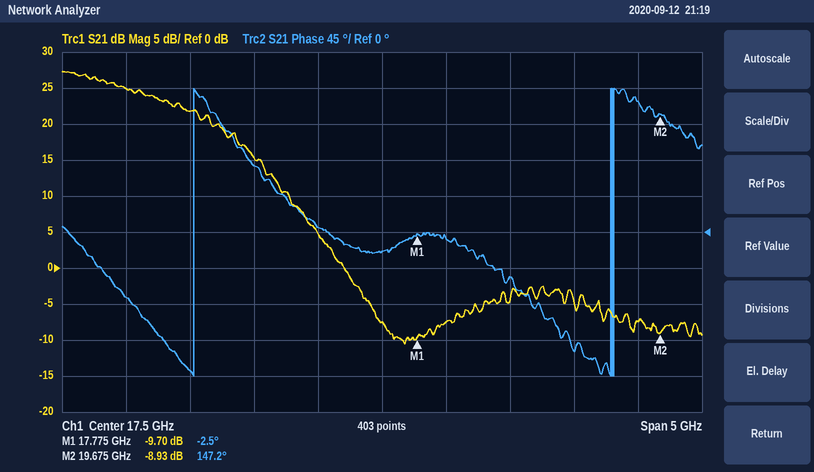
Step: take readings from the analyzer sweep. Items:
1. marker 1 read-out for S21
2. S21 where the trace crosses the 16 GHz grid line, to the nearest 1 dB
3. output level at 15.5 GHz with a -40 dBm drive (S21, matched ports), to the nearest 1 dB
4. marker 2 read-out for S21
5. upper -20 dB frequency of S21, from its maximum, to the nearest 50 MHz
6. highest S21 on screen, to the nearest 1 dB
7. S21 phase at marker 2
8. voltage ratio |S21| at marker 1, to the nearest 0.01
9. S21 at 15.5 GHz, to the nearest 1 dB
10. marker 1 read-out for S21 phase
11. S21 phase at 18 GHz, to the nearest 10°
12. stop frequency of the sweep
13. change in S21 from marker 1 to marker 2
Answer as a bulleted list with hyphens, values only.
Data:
- -9.70 dB
- 22 dB
- -15 dBm
- -8.93 dB
- 16.90 GHz
- 27 dB
- 147.2°
- 0.33
- 25 dB
- -2.5°
- -10°
- 20 GHz
- 0.77 dB
